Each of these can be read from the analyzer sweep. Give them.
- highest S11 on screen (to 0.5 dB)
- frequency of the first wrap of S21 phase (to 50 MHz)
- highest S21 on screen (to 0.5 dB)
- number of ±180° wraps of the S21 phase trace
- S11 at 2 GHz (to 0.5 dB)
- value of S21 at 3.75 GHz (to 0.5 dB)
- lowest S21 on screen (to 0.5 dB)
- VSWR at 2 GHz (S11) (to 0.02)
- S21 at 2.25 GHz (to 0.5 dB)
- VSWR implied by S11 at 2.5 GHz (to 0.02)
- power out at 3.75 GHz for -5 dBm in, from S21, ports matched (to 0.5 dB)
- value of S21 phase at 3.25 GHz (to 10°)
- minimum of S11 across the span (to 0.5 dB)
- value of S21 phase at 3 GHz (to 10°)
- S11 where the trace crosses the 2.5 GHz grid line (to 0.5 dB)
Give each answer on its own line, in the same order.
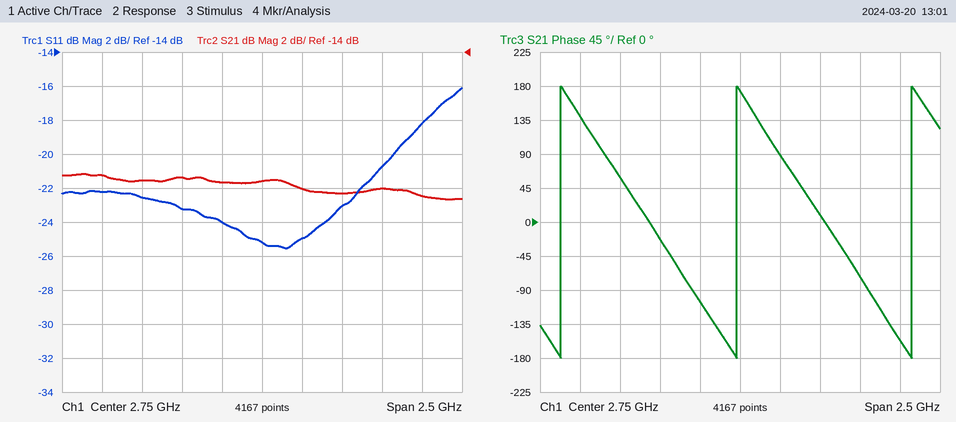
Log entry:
-16.0 dB
1.65 GHz
-21.0 dB
3
-22.5 dB
-22.5 dB
-22.5 dB
1.16
-21.5 dB
1.14
-27.5 dBm
10°
-25.5 dB
90°
-24.0 dB
